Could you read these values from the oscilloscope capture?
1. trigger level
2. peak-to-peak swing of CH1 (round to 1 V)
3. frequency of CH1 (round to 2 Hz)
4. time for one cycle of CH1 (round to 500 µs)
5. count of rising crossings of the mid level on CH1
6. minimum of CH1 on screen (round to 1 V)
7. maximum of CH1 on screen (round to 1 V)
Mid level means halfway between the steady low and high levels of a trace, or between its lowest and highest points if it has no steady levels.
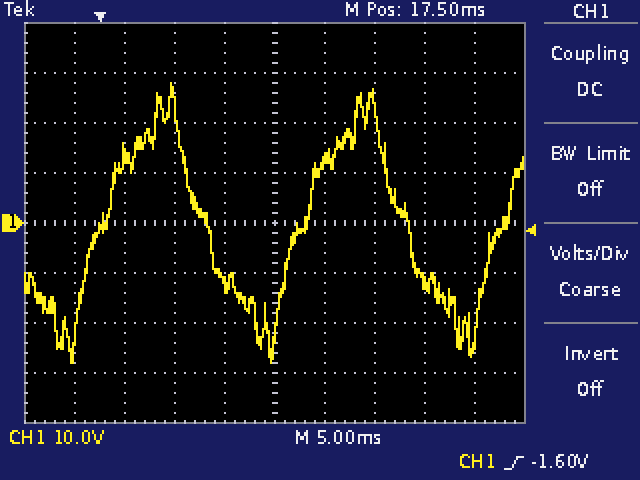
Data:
-1.60 V
56 V
50 Hz
20.0 ms
3
-28 V
28 V
